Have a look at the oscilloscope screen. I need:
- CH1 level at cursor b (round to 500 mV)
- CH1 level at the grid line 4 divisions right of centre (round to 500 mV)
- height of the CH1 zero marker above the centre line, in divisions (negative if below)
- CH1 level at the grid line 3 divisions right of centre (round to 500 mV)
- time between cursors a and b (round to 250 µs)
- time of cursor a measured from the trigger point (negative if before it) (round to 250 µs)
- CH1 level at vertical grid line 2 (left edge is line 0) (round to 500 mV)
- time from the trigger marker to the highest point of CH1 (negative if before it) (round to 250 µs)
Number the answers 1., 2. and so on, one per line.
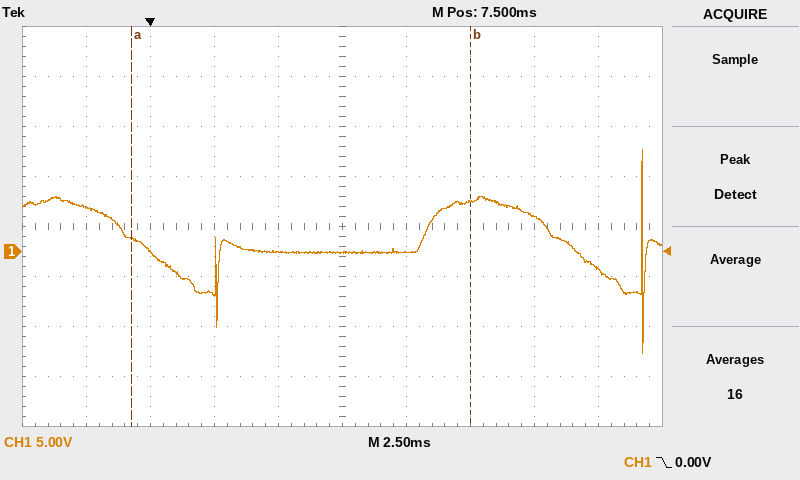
1. 5.0 V
2. -2.0 V
3. -0.5 div
4. 3.5 V
5. 13.25 ms
6. -750 µs
7. 0.0 V
8. +19.25 ms
